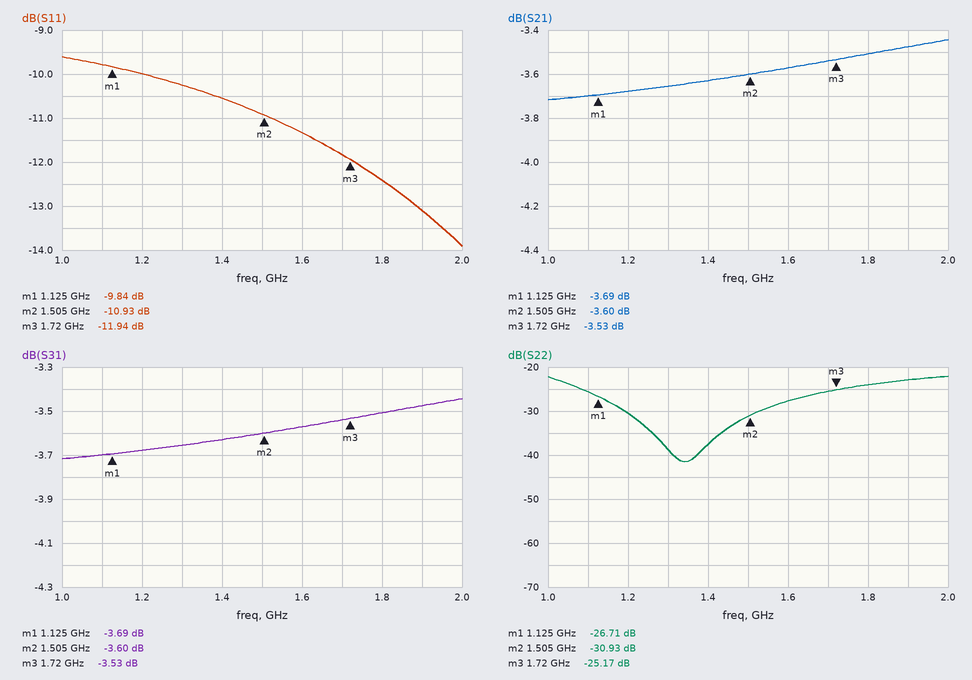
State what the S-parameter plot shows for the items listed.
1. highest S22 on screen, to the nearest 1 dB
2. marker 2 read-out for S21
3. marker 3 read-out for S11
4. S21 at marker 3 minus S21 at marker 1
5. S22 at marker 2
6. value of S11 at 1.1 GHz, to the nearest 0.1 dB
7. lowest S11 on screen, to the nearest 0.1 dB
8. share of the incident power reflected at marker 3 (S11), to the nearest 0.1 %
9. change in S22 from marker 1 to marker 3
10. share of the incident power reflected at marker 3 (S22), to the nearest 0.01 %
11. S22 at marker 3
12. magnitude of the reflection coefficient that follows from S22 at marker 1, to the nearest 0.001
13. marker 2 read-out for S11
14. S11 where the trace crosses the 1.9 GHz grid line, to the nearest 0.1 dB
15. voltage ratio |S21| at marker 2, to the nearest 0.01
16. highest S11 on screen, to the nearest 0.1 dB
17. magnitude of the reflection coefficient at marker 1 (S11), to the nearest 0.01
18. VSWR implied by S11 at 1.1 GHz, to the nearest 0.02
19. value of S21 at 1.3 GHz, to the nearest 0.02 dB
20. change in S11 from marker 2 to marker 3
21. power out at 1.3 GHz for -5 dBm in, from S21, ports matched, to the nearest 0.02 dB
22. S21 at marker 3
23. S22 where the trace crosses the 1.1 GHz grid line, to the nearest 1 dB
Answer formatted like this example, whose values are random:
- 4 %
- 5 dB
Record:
- -22 dB
- -3.60 dB
- -11.94 dB
- 0.16 dB
- -30.93 dB
- -9.8 dB
- -13.9 dB
- 6.4 %
- 1.54 dB
- 0.30 %
- -25.17 dB
- 0.046
- -10.93 dB
- -13.1 dB
- 0.66
- -9.6 dB
- 0.32
- 1.96
- -3.66 dB
- -1.01 dB
- -8.66 dBm
- -3.53 dB
- -26 dB
